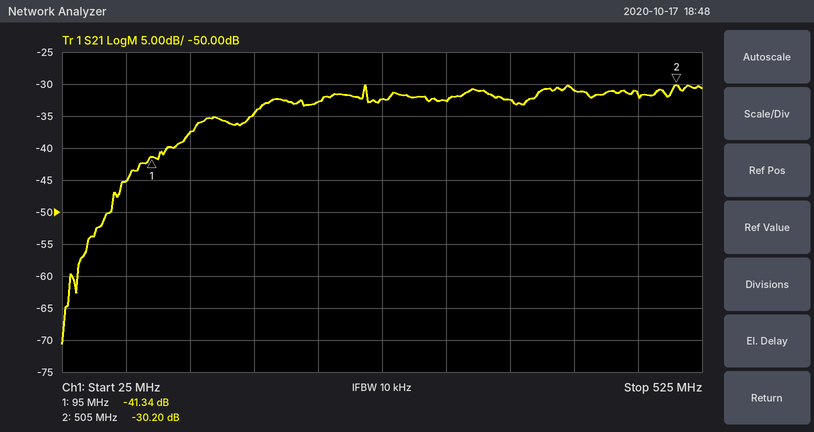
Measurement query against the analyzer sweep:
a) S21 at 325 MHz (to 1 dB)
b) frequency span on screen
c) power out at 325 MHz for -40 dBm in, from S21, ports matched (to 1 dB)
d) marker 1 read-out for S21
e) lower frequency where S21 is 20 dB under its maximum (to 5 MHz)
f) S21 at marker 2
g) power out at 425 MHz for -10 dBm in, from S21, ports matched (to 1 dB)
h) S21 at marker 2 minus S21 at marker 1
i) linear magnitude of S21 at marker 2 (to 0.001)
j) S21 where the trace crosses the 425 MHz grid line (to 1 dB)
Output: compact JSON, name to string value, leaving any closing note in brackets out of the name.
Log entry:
{"S21 at 325 MHz": "-33 dB", "frequency span on screen": "500 MHz", "power out at 325 MHz for -40 dBm in, from S21, ports matched": "-73 dBm", "marker 1 read-out for S21": "-41.34 dB", "lower frequency where S21 is 20 dB under its maximum": "60 MHz", "S21 at marker 2": "-30.20 dB", "power out at 425 MHz for -10 dBm in, from S21, ports matched": "-41 dBm", "S21 at marker 2 minus S21 at marker 1": "11.14 dB", "linear magnitude of S21 at marker 2": "0.031", "S21 where the trace crosses the 425 MHz grid line": "-31 dB"}
